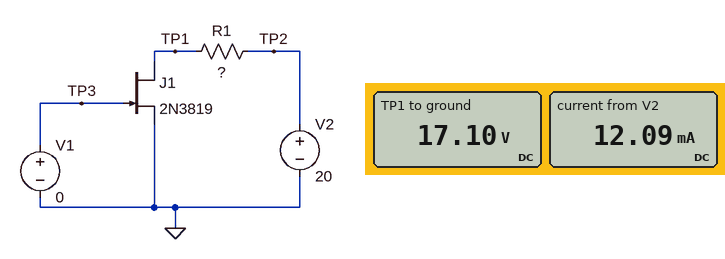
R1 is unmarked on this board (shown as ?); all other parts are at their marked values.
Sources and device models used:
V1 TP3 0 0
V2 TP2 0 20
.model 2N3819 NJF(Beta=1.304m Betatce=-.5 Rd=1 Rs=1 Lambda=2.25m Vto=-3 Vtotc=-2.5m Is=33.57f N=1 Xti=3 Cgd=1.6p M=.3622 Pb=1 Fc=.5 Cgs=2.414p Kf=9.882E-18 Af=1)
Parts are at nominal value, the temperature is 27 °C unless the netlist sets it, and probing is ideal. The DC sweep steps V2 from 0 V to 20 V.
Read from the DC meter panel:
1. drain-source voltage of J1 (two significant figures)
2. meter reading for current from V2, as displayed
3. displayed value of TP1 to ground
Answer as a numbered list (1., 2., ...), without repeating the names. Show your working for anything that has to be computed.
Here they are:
1. 17.1 V = 17 V
2. 12.09 mA
3. 17.10 V
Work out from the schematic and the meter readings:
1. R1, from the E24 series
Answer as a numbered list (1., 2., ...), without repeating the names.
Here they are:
1. 240 Ω
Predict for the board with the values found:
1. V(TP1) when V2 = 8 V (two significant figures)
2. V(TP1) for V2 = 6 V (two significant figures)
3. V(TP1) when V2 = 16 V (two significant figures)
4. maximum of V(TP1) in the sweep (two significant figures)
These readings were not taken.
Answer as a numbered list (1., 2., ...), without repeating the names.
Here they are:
1. 5.2 V
2. 3.2 V
3. 13 V
4. 17 V
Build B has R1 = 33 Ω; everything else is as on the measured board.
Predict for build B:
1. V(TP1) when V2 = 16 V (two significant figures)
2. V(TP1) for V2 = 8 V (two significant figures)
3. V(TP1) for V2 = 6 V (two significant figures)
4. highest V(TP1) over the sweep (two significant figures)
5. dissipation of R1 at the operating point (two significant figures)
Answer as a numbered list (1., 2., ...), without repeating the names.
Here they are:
1. 16 V
2. 7.6 V
3. 5.6 V
4. 20 V
5. 4.9 mW
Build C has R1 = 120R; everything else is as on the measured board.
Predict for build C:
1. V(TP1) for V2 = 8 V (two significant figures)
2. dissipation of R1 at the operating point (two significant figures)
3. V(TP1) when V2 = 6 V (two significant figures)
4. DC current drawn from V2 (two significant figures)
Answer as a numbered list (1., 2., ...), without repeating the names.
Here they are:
1. 6.6 V
2. 18 mW
3. 4.6 V
4. 12 mA
